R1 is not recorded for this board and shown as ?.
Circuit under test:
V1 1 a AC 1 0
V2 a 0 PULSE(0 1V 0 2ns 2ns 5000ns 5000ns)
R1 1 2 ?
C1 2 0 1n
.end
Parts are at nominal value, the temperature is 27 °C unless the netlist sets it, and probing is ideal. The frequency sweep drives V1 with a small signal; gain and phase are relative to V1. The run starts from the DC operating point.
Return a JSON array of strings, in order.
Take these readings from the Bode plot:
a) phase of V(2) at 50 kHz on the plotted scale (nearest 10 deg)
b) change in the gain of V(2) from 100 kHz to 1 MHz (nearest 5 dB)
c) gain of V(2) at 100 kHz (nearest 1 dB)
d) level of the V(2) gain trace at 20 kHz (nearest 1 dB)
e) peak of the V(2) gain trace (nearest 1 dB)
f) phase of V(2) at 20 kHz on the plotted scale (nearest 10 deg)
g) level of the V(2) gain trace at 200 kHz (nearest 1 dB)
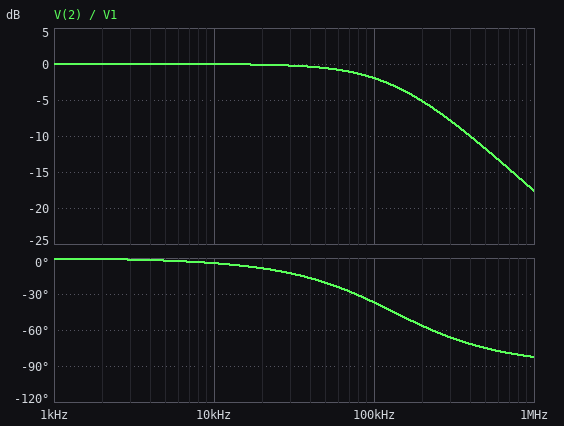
["-20 deg", "-15 dB", "-2 dB", "0 dB", "0 dB", "-10 deg", "-5 dB"]
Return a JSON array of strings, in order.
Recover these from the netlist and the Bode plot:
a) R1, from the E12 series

["1.2 kΩ"]
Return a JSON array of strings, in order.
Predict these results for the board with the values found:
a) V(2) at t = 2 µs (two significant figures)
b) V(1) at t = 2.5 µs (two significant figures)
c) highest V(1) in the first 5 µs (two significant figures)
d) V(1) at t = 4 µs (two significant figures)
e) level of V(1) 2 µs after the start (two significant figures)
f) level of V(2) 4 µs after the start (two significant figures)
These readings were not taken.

["810 mV", "1.0 V", "1.0 V", "1.0 V", "1.0 V", "960 mV"]
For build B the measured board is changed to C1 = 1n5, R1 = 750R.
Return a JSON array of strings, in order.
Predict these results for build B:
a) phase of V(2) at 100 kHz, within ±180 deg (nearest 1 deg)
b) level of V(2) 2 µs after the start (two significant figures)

["-35 deg", "830 mV"]
